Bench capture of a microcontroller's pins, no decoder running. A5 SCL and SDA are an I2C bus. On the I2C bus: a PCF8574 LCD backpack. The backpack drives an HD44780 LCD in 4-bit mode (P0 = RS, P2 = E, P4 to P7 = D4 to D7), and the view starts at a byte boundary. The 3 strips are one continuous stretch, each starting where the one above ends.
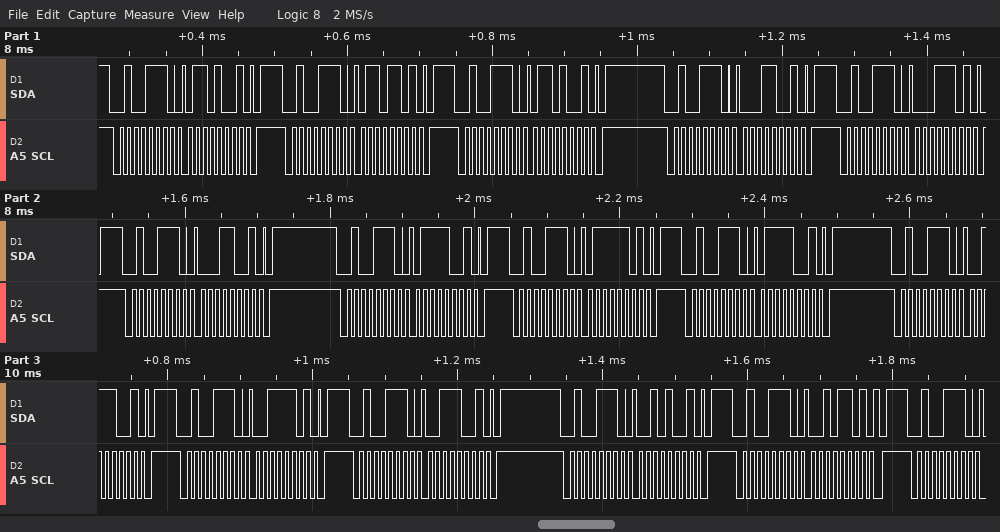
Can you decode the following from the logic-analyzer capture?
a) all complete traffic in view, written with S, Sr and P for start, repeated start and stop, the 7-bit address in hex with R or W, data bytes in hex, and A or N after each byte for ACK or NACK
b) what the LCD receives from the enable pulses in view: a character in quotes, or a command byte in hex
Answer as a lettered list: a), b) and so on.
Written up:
a) S 27W A 69 A P S 27W A 6D A P S 27W A 69 A P S 27W A 19 A P S 27W A 1D A P S 27W A 19 A P S 27W A 79 A P S 27W A 7D A P S 27W A 79 A P S 27W A 39 A P S 27W A 3D A P S 27W A 39 A P S 27W A 29 A P S 27W A 2D A P S 27W A
b) 'a' 's'
